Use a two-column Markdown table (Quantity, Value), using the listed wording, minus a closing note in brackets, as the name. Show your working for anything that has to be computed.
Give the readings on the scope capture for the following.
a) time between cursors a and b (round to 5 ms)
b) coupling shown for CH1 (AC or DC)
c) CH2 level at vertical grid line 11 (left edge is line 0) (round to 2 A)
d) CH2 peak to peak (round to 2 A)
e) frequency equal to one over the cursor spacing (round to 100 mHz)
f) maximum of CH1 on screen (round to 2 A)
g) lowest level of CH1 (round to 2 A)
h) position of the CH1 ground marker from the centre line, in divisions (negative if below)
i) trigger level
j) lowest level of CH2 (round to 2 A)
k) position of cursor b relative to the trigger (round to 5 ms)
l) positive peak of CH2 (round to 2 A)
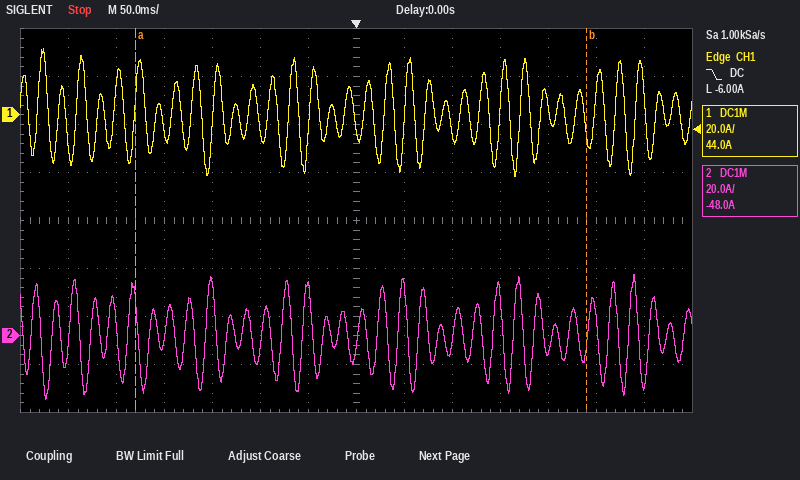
| Quantity | Value |
|---|---|
| time between cursors a and b | 470 ms |
| coupling shown for CH1 | DC |
| CH2 level at vertical grid line 11 (left edge is line 0) | -6 A |
| CH2 peak to peak | 26 A − (-26 A) = 52 A |
| frequency equal to one over the cursor spacing | 1 / 470 ms ≈ 2.1 Hz |
| maximum of CH1 on screen | 28 A |
| lowest level of CH1 | -26 A |
| position of the CH1 ground marker from the centre line, in divisions | +2.2 div |
| trigger level | -6.00 A |
| lowest level of CH2 | -26 A |
| position of cursor b relative to the trigger | +240 ms |
| positive peak of CH2 | 26 A |
